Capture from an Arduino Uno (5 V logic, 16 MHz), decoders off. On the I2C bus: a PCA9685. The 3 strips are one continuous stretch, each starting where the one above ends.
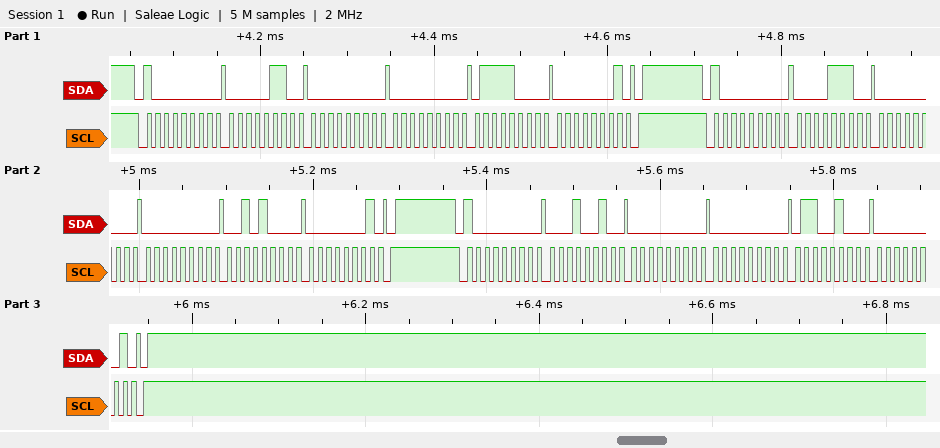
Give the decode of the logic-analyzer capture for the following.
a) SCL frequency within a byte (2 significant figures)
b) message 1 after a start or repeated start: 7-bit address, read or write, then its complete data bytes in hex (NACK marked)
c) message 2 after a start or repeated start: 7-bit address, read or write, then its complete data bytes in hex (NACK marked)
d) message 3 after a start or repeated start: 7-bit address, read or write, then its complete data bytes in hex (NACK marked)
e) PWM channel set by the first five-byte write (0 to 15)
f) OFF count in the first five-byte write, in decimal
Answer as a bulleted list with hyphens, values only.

- 100 kHz
- 0x40 write: 06 00 00 78 01
- 0x40 write: 0E 00 00 28 01
- 0x40 write: 12 00 00 64 01
- 0
- 376
